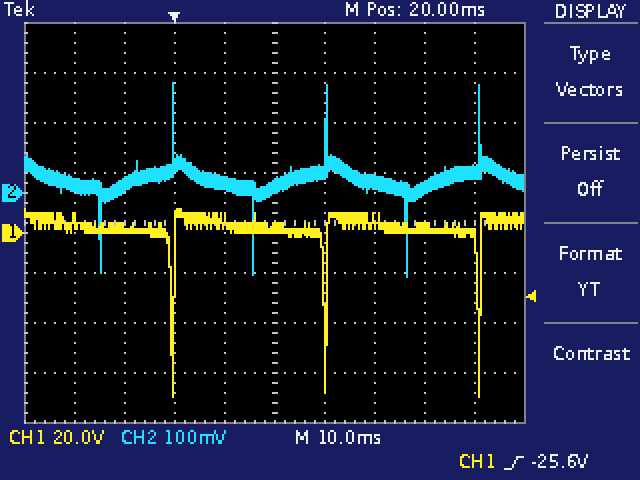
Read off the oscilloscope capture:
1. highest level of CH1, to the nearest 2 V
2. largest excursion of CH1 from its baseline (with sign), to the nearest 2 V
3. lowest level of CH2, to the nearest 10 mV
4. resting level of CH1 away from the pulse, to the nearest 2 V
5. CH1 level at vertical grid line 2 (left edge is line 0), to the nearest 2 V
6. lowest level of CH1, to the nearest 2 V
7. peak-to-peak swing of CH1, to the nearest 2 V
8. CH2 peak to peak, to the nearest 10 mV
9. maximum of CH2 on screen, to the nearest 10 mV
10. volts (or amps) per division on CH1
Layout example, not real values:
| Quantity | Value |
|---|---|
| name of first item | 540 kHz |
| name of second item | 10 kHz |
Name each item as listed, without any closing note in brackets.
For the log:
| Quantity | Value |
|---|---|
| highest level of CH1, to the nearest 2 V | 10 V |
| largest excursion of CH1 from its baseline (with sign), to the nearest 2 V | -68 V |
| lowest level of CH2, to the nearest 10 mV | -170 mV |
| resting level of CH1 away from the pulse, to the nearest 2 V | 2 V |
| CH1 level at vertical grid line 2 (left edge is line 0), to the nearest 2 V | 2 V |
| lowest level of CH1, to the nearest 2 V | -66 V |
| peak-to-peak swing of CH1, to the nearest 2 V | 76 V |
| CH2 peak to peak, to the nearest 10 mV | 390 mV |
| maximum of CH2 on screen, to the nearest 10 mV | 220 mV |
| volts (or amps) per division on CH1 | 20 V |
